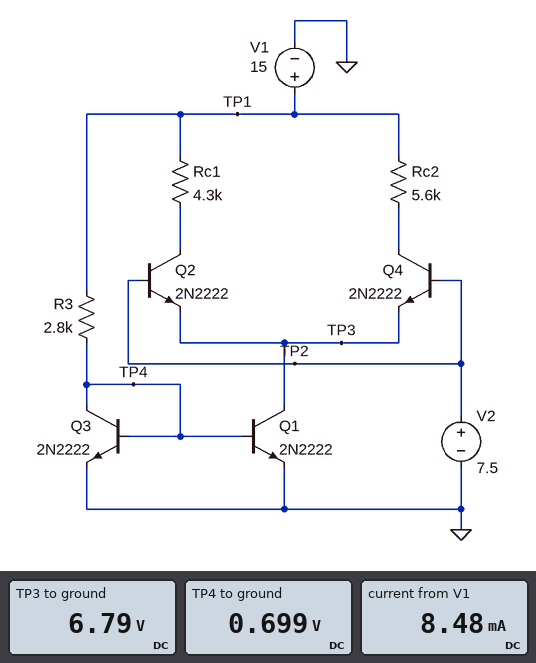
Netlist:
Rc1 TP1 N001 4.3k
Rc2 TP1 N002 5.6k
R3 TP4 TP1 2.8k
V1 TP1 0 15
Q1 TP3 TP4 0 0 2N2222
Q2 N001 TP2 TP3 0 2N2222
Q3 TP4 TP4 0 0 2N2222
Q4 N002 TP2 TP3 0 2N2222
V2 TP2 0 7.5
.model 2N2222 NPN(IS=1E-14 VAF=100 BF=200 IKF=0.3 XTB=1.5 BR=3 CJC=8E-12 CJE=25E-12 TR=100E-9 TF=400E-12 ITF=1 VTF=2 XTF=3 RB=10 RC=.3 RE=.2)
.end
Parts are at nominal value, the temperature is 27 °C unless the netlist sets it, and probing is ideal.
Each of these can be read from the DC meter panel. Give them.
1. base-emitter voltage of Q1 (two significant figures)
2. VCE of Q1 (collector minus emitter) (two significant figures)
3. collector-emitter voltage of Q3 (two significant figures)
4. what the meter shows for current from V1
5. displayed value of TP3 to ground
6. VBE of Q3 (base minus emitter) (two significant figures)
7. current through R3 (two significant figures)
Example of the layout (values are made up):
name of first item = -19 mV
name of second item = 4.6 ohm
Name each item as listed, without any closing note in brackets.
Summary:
base-emitter voltage of Q1 = 700 mV
VCE of Q1 (collector minus emitter) = 6.8 V
collector-emitter voltage of Q3 = 700 mV
what the meter shows for current from V1 = 8.48 mA
displayed value of TP3 to ground = 6.79 V
VBE of Q3 (base minus emitter) = 700 mV
current through R3 = 5.1 mA
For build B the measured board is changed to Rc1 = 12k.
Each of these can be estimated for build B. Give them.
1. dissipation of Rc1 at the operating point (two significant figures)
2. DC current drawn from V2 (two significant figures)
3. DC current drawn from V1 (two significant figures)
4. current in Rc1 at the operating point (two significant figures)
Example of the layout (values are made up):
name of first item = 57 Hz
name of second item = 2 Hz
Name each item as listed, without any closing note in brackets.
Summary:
dissipation of Rc1 at the operating point = 5.6 mW
DC current drawn from V2 = 3.2 mA
DC current drawn from V1 = 7.3 mA
current in Rc1 at the operating point = 680 µA
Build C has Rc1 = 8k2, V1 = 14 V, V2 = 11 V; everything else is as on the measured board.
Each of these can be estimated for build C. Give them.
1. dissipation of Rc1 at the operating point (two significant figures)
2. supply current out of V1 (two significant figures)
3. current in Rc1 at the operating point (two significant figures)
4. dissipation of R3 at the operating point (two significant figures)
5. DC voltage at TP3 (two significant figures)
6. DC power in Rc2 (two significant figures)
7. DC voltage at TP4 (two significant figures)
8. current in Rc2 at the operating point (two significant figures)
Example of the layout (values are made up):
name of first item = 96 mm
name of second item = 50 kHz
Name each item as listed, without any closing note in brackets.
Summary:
dissipation of Rc1 at the operating point = 1.7 mW
supply current out of V1 = 5.9 mA
current in Rc1 at the operating point = 450 µA
dissipation of R3 at the operating point = 63 mW
DC voltage at TP3 = 10 V
DC power in Rc2 = 2.5 mW
DC voltage at TP4 = 700 mV
current in Rc2 at the operating point = 660 µA
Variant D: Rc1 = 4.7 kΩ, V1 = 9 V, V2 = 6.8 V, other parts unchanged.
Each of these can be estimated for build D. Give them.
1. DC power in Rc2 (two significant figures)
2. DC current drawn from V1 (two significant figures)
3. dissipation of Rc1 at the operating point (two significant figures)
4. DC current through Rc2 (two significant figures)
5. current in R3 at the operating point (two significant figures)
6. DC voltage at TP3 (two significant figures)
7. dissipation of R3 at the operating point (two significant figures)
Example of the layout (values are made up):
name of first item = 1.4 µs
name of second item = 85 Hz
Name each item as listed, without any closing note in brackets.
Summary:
DC power in Rc2 = 1.5 mW
DC current drawn from V1 = 4.1 mA
dissipation of Rc1 at the operating point = 1.8 mW
DC current through Rc2 = 520 µA
current in R3 at the operating point = 3.0 mA
DC voltage at TP3 = 6.1 V
dissipation of R3 at the operating point = 25 mW
